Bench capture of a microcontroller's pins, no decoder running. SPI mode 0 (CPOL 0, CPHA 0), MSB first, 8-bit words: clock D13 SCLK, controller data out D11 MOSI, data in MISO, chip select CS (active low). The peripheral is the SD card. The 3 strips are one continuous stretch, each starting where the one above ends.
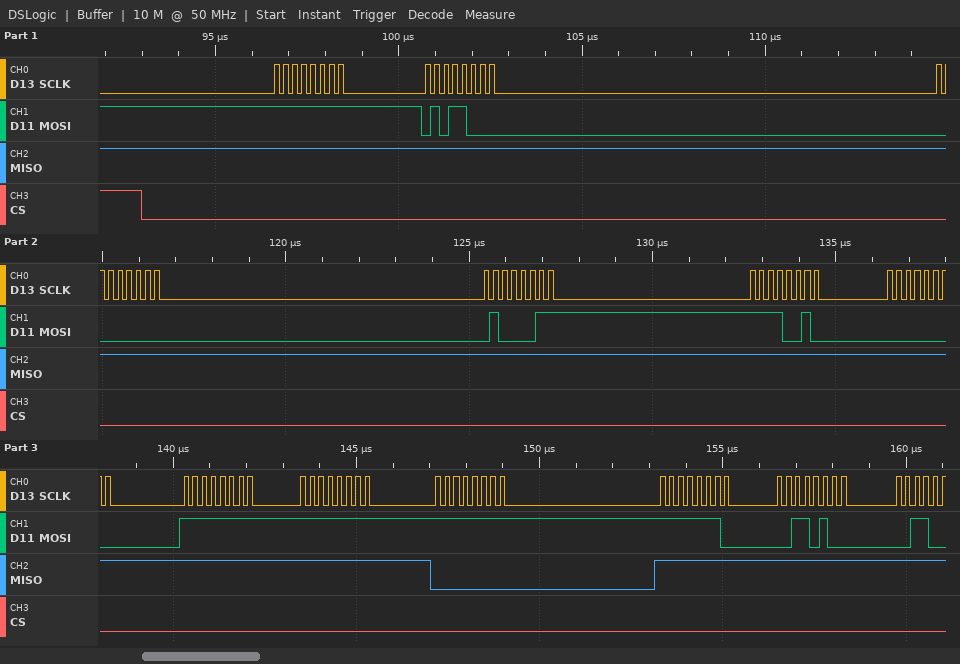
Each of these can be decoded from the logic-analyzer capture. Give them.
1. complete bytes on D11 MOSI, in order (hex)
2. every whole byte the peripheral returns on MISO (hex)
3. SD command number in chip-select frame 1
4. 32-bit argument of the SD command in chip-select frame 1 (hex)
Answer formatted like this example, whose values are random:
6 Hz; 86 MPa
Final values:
FF 58 00 43 F2 00 FF FF FF FE 34; FF FF FF FF FF FF FF FF 00 FF FF; CMD24; 0x0043F200
